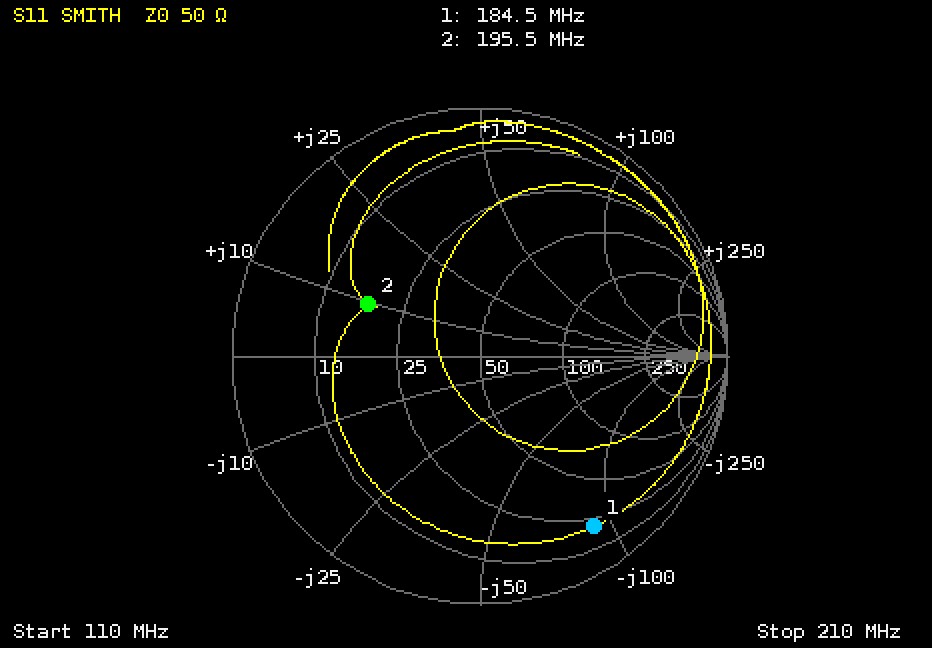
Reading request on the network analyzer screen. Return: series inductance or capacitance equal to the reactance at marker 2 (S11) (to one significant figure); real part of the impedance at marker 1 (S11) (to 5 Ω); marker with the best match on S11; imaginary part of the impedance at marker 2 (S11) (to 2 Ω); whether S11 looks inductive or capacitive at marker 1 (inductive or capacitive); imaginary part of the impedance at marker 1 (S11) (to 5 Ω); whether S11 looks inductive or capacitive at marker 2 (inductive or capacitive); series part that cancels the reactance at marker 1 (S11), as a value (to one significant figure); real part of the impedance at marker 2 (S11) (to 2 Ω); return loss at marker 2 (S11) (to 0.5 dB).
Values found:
8 nH
20 Ω
marker 2
+10 Ω
capacitive
-90 Ω
inductive
80 nH
18 Ω
6.0 dB
